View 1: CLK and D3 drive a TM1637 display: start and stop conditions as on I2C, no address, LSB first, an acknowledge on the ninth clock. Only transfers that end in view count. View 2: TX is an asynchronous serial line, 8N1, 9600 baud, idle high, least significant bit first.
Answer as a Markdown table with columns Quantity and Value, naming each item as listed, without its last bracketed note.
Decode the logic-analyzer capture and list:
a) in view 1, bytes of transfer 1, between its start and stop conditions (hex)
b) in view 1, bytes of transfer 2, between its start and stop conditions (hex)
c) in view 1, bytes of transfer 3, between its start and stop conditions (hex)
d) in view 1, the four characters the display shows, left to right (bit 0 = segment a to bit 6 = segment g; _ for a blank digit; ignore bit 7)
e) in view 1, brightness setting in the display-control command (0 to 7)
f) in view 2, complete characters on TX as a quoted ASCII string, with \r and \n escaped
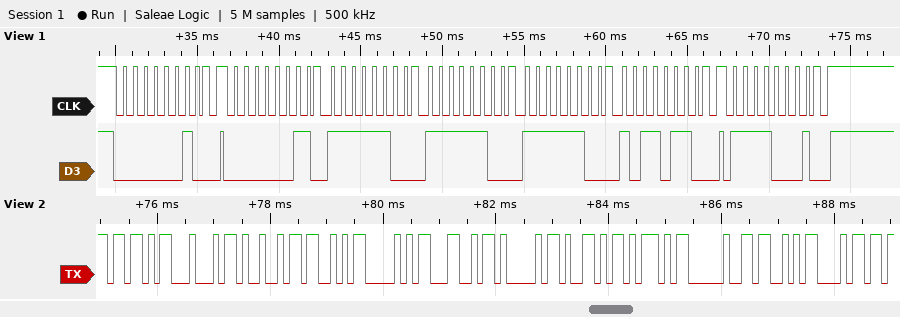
| Quantity | Value |
|---|---|
| in view 1, bytes of transfer 1, between its start and stop conditions | 40 |
| in view 1, bytes of transfer 2, between its start and stop conditions | C0 3F 3F 3F 6D |
| in view 1, bytes of transfer 3, between its start and stop conditions | 8F |
| in view 1, the four characters the display shows, left to right | 0005 |
| in view 1, brightness setting in the display-control command | 7 |
| in view 2, complete characters on TX as a quoted ASCII string, with \r and \n escaped | "[DISPLAY] Sh" |
